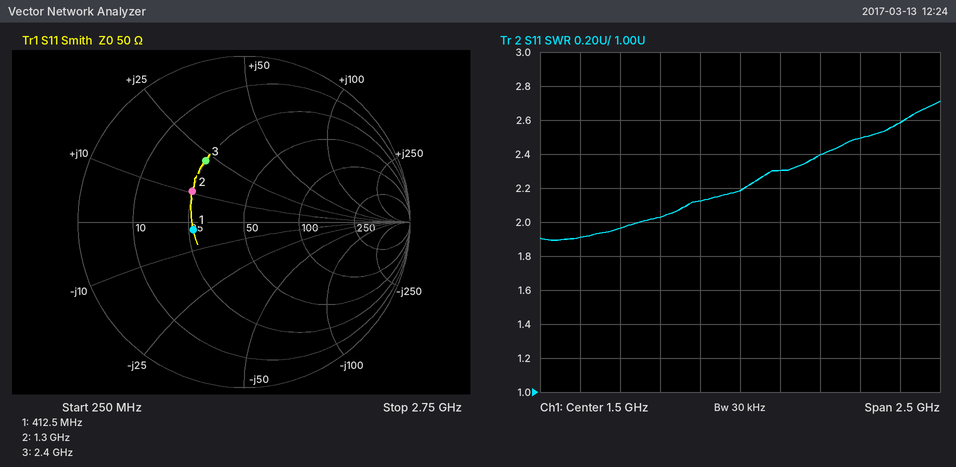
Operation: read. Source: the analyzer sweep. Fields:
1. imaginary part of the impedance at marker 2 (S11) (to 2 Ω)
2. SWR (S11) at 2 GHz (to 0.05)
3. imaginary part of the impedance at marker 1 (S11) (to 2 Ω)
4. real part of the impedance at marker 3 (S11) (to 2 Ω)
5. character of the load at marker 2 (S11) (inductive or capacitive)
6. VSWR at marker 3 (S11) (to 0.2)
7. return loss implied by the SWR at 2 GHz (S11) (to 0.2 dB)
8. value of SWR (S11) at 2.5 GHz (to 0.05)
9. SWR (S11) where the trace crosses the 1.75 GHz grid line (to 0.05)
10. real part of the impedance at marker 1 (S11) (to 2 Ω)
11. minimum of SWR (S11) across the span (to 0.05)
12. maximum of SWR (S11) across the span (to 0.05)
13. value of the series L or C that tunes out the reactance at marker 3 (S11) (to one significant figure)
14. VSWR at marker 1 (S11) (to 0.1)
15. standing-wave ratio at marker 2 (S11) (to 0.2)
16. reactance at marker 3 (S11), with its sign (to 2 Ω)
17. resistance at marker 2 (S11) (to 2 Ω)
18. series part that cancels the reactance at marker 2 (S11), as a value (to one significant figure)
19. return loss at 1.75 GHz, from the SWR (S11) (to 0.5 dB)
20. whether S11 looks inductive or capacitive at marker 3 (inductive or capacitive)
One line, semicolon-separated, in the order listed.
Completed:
+10 Ω; 2.40; -2 Ω; 24 Ω; inductive; 2.6; 7.8 dB; 2.60; 2.30; 26 Ω; 1.90; 2.70; 3 pF; 1.9; 2.2; +22 Ω; 24 Ω; 10 pF; 8.0 dB; inductive
